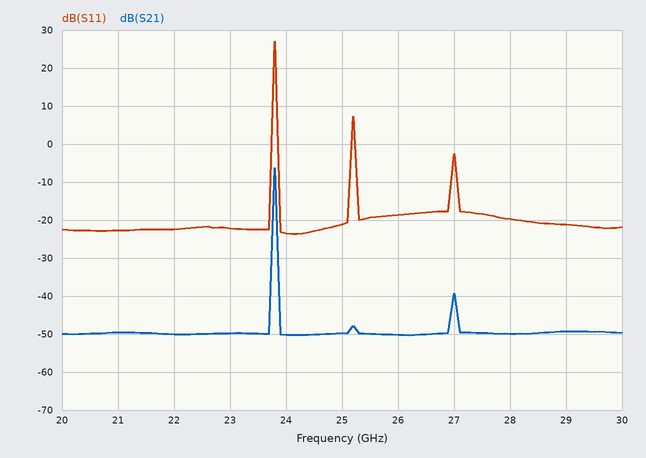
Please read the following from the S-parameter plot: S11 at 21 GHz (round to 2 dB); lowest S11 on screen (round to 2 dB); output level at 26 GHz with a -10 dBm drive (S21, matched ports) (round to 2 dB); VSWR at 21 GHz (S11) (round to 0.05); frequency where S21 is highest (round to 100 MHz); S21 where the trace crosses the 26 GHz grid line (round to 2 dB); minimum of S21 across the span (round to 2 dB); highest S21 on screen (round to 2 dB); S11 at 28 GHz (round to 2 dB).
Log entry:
-22 dB
-24 dB
-60 dBm
1.15
23.8 GHz
-50 dB
-50 dB
-6 dB
-20 dB
